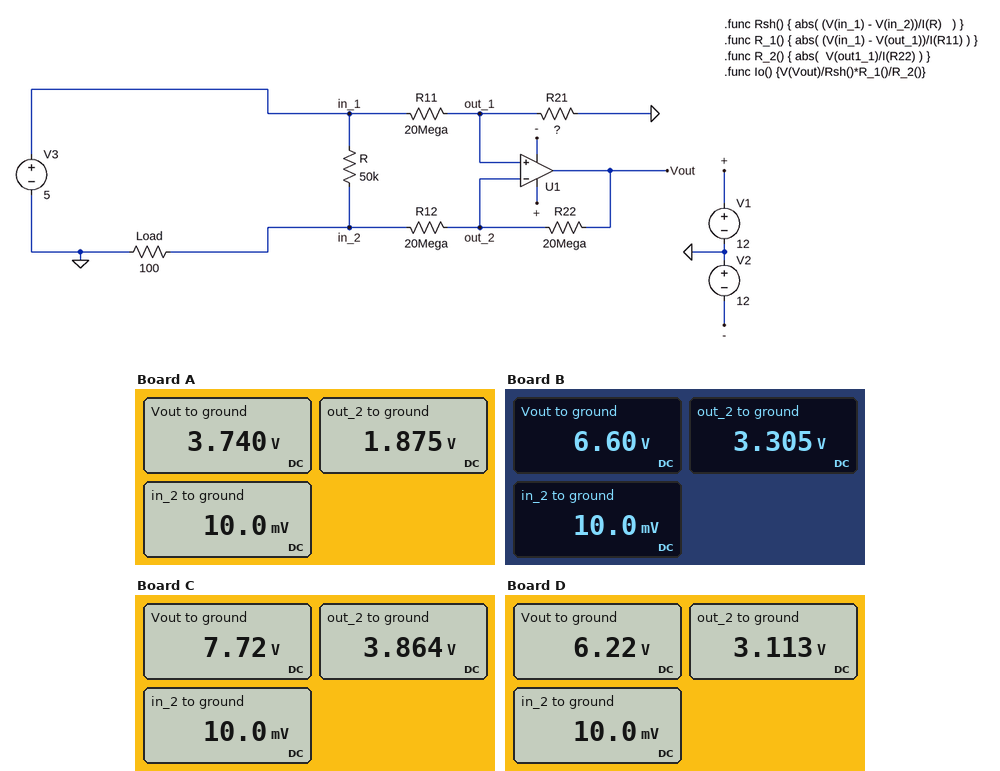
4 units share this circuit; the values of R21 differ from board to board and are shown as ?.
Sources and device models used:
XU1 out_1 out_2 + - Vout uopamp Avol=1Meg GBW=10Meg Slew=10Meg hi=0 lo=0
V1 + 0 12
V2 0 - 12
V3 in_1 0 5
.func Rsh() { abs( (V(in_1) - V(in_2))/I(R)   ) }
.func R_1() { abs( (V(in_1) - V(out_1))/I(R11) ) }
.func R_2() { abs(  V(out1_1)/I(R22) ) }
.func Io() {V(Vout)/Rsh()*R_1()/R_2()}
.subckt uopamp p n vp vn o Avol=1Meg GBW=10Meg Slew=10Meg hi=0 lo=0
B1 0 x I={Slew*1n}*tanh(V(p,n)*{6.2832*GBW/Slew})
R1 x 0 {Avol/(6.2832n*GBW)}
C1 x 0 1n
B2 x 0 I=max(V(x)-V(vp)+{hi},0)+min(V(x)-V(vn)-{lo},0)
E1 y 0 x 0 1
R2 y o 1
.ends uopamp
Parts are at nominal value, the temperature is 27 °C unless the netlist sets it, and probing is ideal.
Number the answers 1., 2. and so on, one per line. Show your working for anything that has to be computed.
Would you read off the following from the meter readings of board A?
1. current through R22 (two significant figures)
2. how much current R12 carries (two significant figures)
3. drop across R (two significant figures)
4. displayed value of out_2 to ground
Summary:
1. (3.74 V - 1.875 V) / 20 MΩ = 93 nA
2. (1.875 V - 10 mV) / 20 MΩ = 93 nA
3. 5 V - 10 mV = 5.0 V
4. 1.875 V
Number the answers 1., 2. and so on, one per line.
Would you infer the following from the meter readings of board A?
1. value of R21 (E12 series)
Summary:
1. 12 MΩ
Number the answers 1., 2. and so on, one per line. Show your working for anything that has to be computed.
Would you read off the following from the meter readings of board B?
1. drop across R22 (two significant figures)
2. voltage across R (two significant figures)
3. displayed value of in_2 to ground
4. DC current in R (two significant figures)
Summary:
1. 6.6 V - 3.305 V = 3.3 V
2. 5 V - 10 mV = 5.0 V
3. 10.0 mV
4. (5 V - 10 mV) / 50 kΩ = 100 µA
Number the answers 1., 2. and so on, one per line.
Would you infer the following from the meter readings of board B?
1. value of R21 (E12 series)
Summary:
1. 39 MΩ
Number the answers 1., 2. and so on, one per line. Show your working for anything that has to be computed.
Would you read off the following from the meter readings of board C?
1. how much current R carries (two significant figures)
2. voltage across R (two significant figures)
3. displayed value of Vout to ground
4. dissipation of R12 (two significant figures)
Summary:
1. (5 V - 10 mV) / 50 kΩ = 100 µA
2. 5 V - 10 mV = 5.0 V
3. 7.72 V
4. (3.864 V - 10 mV)^2 / 20 MΩ = 740 nW
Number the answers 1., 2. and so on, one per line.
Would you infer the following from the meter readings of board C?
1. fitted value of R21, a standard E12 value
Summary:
1. 68 MΩ
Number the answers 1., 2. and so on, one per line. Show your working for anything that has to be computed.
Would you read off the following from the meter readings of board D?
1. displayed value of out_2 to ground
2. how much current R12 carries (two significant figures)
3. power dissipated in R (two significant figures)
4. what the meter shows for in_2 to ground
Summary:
1. 3.113 V
2. (3.113 V - 10 mV) / 20 MΩ = 160 nA
3. (5 V - 10 mV)^2 / 50 kΩ = 500 µW
4. 10.0 mV
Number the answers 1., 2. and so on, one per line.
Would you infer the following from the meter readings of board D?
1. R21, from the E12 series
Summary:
1. 33 MΩ
